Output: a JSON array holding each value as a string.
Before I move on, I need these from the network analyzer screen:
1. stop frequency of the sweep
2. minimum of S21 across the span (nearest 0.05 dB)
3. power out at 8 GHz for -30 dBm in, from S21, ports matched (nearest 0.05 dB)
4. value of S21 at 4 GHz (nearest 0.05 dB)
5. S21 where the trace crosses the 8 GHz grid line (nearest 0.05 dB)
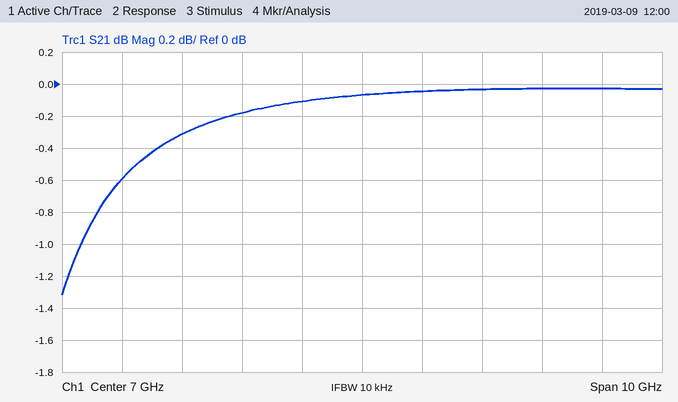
["12 GHz", "-1.30 dB", "-30.05 dBm", "-0.30 dB", "-0.05 dB"]
